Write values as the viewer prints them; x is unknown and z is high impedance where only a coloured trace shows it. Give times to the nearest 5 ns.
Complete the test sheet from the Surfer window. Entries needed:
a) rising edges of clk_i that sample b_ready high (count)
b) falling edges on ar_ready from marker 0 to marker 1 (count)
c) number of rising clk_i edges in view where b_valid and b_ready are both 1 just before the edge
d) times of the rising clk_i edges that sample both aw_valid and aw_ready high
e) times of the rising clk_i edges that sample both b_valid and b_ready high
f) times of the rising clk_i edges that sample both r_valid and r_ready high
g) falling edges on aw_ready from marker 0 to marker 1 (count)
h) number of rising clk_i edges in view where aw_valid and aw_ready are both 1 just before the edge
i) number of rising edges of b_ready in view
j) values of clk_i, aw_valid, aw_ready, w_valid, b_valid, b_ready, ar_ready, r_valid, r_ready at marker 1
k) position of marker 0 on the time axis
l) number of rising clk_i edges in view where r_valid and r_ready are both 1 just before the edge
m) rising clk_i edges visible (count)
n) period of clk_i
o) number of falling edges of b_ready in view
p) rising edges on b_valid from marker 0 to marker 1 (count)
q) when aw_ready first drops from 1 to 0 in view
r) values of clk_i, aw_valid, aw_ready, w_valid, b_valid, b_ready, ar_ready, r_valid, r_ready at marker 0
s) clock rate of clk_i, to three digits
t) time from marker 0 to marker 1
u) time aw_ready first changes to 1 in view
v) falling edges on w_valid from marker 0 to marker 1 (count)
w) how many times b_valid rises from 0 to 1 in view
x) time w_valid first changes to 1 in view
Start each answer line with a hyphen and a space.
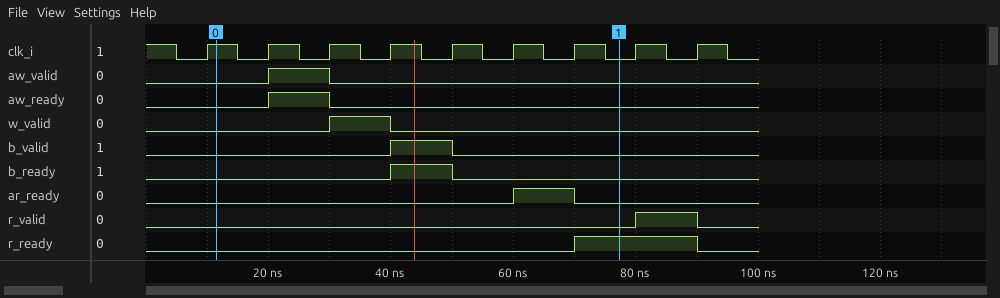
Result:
- 1
- 1
- 1
- 30 ns
- 50 ns
- 90 ns
- 1
- 1
- 1
- clk_i=0, aw_valid=0, aw_ready=0, w_valid=0, b_valid=0, b_ready=0, ar_ready=0, r_valid=0, r_ready=1
- 10 ns
- 1
- 9
- 10 ns
- 1
- 1
- 30 ns
- clk_i=1, aw_valid=0, aw_ready=0, w_valid=0, b_valid=0, b_ready=0, ar_ready=0, r_valid=0, r_ready=0
- 100 MHz
- 65 ns
- 20 ns
- 1
- 1
- 30 ns
